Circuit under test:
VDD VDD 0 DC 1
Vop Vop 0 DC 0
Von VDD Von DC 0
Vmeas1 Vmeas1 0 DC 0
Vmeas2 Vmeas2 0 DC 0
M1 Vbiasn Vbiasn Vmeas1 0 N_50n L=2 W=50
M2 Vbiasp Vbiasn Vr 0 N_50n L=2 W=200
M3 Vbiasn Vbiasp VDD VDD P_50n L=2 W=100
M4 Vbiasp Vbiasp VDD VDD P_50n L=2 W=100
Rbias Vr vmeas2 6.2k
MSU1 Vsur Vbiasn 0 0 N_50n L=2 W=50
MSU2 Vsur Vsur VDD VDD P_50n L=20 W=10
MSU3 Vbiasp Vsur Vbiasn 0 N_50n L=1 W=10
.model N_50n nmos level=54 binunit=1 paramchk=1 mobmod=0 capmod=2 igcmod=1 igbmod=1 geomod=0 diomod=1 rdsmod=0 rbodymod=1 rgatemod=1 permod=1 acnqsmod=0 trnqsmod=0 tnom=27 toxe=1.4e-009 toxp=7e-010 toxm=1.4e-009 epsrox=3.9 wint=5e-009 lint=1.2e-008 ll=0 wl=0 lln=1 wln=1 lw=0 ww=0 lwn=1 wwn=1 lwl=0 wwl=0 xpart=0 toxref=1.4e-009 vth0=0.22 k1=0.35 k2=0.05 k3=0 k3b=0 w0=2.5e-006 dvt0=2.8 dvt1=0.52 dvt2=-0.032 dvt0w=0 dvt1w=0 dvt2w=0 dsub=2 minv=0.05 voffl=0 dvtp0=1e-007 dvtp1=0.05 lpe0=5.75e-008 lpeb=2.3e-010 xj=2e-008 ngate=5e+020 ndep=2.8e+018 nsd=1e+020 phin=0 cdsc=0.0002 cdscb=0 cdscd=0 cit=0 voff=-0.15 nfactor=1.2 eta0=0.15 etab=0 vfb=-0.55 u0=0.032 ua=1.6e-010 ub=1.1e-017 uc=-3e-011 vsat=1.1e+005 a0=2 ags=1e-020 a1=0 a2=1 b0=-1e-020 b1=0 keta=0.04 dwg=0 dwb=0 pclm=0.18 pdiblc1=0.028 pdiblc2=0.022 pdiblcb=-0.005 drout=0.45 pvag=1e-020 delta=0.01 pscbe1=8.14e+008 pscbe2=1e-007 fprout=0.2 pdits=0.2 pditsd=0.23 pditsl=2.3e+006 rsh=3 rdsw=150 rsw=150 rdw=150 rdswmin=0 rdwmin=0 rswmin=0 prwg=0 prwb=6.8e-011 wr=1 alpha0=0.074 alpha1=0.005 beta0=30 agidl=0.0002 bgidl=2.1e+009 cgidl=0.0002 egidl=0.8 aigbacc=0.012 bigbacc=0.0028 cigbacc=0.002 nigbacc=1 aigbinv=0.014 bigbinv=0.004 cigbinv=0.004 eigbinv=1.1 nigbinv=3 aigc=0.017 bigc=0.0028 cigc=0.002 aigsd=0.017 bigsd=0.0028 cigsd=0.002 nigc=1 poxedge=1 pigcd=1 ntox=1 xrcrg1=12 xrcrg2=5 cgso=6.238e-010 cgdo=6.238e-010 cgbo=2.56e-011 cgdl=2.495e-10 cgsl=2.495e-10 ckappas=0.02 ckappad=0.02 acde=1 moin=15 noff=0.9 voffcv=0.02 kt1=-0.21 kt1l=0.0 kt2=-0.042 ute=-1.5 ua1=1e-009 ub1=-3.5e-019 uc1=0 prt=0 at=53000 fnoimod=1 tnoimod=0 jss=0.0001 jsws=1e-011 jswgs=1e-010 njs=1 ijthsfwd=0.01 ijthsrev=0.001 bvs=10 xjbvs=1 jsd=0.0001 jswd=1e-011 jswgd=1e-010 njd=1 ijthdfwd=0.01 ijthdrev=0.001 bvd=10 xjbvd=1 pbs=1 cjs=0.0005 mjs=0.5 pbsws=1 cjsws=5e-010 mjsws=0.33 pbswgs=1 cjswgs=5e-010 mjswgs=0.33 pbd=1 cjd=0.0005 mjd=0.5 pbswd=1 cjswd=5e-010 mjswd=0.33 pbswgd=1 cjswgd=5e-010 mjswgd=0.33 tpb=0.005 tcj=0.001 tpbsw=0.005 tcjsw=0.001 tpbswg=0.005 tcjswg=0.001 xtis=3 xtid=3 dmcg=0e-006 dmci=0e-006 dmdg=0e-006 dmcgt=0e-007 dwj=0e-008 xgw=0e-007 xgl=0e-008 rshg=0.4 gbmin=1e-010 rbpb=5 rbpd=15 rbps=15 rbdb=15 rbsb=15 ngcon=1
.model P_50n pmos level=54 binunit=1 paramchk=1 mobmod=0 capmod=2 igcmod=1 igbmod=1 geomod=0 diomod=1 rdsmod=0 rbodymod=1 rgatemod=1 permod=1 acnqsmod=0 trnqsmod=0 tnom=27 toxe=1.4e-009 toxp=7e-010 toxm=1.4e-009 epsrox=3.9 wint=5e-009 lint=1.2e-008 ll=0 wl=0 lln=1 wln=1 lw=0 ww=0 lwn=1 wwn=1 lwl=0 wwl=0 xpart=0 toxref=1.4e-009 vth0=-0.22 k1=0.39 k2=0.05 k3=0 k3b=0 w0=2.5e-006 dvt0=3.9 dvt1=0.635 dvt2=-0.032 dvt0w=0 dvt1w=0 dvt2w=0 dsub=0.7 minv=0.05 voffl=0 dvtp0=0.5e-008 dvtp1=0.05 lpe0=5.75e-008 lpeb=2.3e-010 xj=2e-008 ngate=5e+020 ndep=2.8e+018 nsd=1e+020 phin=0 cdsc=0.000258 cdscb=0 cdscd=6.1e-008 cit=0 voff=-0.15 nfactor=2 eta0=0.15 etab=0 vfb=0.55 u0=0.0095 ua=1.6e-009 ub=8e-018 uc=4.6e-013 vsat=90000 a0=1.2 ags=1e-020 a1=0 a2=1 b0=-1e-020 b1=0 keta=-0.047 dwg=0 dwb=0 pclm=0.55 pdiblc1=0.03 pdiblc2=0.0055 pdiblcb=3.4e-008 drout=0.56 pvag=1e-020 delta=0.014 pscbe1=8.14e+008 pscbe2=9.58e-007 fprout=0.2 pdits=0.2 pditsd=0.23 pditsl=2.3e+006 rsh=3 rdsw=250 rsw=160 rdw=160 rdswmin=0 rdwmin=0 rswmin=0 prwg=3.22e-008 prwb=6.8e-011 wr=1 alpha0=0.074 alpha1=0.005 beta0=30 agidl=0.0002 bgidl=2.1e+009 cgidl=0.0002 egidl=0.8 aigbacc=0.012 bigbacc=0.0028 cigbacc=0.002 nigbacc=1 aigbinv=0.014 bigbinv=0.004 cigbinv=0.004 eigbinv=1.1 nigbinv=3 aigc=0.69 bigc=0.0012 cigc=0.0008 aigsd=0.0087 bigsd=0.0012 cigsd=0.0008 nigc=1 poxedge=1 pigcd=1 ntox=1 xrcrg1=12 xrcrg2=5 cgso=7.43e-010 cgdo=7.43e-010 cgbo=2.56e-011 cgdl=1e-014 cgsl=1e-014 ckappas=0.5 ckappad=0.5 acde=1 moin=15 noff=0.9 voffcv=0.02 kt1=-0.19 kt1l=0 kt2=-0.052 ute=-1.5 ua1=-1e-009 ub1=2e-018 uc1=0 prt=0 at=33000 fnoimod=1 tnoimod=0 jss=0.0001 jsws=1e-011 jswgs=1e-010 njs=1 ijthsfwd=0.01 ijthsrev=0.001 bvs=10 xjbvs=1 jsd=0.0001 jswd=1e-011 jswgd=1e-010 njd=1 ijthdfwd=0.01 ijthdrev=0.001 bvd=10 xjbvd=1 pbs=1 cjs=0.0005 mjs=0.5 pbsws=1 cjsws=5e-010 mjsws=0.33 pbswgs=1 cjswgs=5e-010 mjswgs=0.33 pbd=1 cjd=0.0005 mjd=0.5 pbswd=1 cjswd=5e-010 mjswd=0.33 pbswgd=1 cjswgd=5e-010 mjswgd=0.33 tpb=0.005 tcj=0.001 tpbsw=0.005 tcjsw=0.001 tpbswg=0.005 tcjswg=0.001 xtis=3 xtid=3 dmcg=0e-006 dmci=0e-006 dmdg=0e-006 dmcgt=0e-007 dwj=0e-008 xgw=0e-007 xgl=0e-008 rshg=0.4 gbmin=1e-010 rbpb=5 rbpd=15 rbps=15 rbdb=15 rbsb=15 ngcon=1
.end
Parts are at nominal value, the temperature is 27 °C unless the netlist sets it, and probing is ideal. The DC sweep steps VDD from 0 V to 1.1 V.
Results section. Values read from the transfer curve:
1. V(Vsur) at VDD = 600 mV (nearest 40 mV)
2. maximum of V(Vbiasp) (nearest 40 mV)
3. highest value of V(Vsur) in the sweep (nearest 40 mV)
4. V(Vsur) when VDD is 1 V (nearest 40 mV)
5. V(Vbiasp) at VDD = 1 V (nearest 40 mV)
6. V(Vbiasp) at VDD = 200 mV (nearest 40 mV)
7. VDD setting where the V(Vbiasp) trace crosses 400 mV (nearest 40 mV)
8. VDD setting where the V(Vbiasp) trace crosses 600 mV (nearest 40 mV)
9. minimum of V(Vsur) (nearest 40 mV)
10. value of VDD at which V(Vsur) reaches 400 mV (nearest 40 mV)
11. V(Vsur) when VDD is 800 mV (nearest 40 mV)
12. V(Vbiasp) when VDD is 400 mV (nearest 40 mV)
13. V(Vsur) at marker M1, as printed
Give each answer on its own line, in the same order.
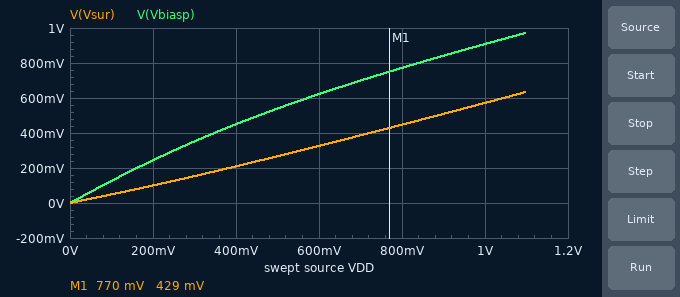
320 mV
960 mV
640 mV
560 mV
920 mV
240 mV
360 mV
560 mV
0 V
720 mV
440 mV
440 mV
429 mV
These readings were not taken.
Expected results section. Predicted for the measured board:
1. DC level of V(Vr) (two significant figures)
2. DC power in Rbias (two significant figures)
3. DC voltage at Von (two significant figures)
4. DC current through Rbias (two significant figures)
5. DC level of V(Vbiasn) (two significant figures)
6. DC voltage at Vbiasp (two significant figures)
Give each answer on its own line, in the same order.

220 mV
8.0 µW
1.0 V
36 µA
320 mV
910 mV
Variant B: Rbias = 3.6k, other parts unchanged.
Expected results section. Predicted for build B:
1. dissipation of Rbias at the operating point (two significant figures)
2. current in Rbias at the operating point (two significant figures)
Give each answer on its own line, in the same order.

14 µW
62 µA
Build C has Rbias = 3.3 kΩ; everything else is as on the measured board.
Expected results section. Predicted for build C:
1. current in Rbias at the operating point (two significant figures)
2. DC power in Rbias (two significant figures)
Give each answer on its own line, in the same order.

67 µA
15 µW
